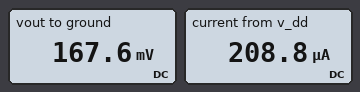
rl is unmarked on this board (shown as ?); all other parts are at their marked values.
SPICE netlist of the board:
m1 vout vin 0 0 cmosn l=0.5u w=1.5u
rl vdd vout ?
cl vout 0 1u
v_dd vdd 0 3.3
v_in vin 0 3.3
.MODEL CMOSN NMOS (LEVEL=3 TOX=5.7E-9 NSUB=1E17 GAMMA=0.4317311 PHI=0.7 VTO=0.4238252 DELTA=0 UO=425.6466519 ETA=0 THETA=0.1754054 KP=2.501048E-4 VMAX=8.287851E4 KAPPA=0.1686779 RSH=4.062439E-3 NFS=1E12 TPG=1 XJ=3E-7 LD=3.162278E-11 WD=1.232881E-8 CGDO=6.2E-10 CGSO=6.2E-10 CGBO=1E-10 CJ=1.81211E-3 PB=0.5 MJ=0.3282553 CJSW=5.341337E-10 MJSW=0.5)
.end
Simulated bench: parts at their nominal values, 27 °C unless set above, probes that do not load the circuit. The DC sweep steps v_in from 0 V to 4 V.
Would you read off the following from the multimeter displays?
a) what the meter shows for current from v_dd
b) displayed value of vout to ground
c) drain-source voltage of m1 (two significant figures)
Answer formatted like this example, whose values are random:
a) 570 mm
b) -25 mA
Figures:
a) 208.8 µA
b) 167.6 mV
c) 170 mV
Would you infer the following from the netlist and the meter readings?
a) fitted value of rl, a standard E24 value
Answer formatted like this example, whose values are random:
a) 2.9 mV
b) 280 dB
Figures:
a) 15 kΩ
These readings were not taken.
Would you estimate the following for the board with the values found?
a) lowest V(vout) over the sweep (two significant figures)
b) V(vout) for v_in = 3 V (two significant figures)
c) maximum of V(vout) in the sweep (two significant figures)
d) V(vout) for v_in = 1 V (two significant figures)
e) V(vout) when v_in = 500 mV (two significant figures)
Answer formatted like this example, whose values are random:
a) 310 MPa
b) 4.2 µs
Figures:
a) 140 mV
b) 180 mV
c) 3.3 V
d) 1.9 V
e) 3.2 V
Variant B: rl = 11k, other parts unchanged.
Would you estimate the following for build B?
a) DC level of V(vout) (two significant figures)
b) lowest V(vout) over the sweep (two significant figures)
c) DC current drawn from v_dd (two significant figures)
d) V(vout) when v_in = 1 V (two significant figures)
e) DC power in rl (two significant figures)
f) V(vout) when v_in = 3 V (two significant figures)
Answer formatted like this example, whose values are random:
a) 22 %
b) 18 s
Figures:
a) 240 mV
b) 200 mV
c) 280 µA
d) 2.3 V
e) 850 µW
f) 260 mV
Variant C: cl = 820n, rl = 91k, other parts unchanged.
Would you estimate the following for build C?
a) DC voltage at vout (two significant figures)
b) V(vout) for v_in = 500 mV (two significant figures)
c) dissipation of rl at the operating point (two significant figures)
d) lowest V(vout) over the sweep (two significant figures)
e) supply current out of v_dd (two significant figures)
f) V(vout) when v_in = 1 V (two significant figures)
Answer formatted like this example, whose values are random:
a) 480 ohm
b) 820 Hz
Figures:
a) 26 mV
b) 2.7 V
c) 120 µW
d) 22 mV
e) 36 µA
f) 98 mV
